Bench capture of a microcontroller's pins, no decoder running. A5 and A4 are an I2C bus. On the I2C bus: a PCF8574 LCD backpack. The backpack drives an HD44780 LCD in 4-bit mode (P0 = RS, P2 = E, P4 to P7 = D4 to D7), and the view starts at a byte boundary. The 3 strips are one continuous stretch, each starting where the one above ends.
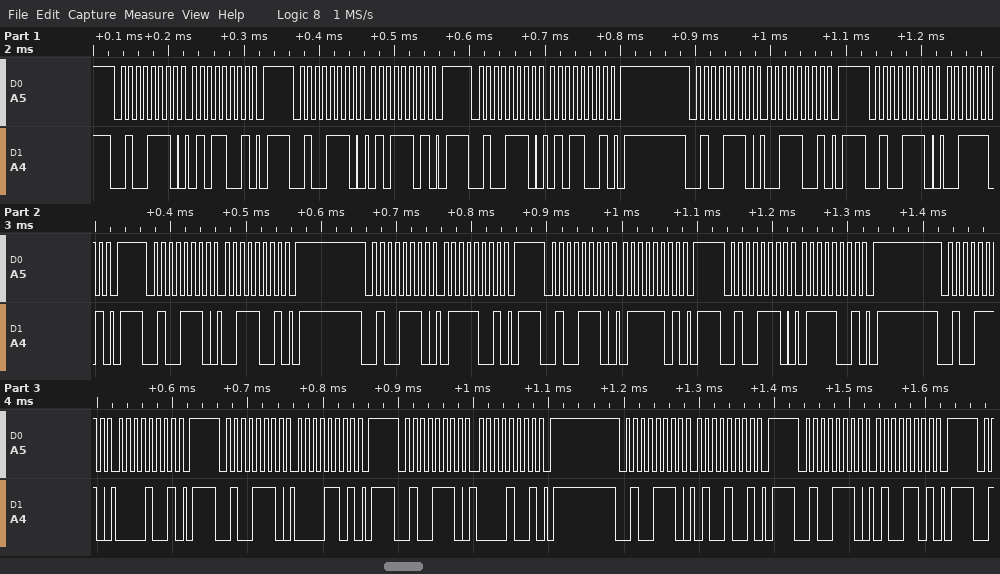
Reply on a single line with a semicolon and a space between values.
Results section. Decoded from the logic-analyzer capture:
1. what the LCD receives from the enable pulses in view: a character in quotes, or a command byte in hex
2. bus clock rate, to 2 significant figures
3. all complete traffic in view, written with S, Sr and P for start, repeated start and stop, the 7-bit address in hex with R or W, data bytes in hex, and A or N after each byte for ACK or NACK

'S' 'p'; 100 kHz; S 27W A 59 A P S 27W A 5D A P S 27W A 59 A P S 27W A 39 A P S 27W A 3D A P S 27W A 39 A P S 27W A 79 A P S 27W A 7D A P S 27W A 79 A P S 27W A 09 A P S 27W A 0D A P S 27W A 09 A P S 27W A 49 A P S 27W A 4D A P
